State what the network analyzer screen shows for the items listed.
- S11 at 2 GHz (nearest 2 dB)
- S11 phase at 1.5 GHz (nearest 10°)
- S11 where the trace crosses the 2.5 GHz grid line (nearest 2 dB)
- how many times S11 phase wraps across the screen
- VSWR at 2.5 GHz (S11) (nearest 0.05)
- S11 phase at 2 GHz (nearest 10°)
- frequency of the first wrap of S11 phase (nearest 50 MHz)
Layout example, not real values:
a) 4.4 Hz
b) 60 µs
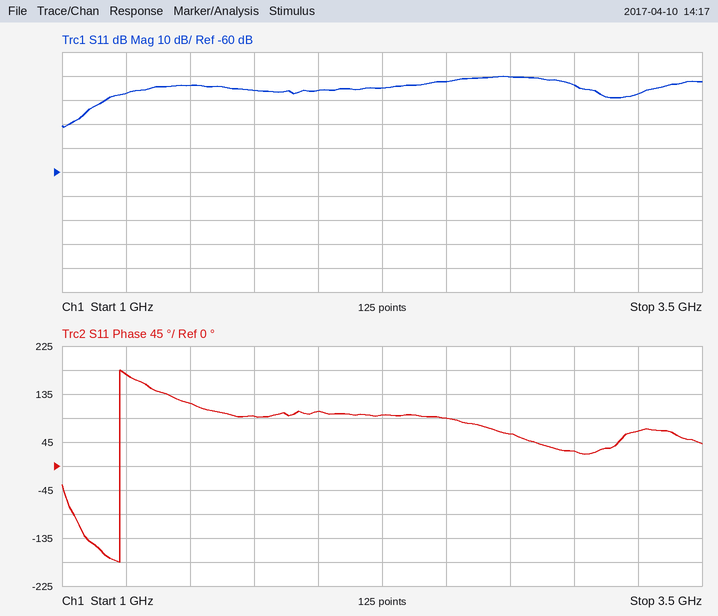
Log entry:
a) -26 dB
b) 120°
c) -22 dB
d) 1
e) 1.15
f) 100°
g) 1.20 GHz
